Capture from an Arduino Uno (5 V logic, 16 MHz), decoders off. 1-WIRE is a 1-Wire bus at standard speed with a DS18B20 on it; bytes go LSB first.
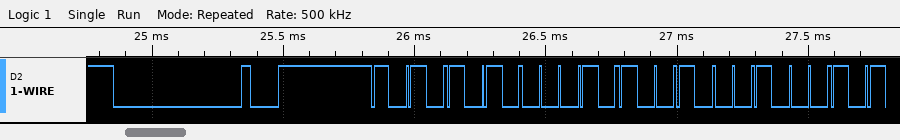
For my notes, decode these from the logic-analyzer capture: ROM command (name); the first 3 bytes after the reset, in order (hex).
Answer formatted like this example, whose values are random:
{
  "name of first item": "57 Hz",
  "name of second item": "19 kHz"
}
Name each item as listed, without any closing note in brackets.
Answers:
{
  "ROM command": "Match ROM",
  "the first 3 bytes after the reset, in order": "55 28 11"
}
